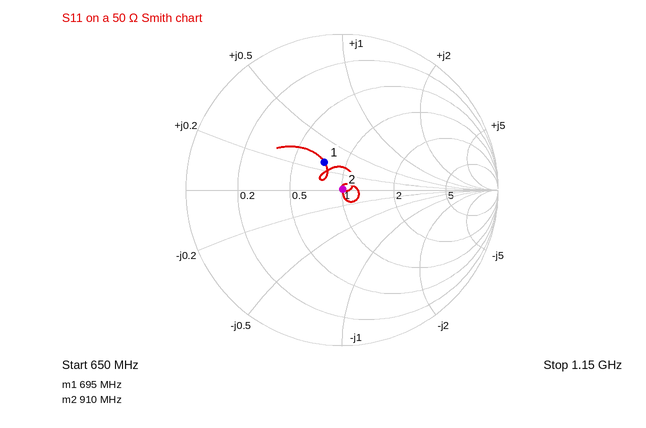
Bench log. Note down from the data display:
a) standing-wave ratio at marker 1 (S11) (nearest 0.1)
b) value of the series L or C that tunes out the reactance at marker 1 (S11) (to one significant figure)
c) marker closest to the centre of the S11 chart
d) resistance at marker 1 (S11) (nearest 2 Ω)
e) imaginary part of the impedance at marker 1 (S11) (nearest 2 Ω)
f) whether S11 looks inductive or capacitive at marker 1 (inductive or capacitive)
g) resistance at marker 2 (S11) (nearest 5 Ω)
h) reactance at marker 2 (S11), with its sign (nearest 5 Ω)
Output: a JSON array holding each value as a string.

["1.5", "20 pF", "marker 2", "38 Ω", "+14 Ω", "inductive", "50 Ω", "0 Ω"]
